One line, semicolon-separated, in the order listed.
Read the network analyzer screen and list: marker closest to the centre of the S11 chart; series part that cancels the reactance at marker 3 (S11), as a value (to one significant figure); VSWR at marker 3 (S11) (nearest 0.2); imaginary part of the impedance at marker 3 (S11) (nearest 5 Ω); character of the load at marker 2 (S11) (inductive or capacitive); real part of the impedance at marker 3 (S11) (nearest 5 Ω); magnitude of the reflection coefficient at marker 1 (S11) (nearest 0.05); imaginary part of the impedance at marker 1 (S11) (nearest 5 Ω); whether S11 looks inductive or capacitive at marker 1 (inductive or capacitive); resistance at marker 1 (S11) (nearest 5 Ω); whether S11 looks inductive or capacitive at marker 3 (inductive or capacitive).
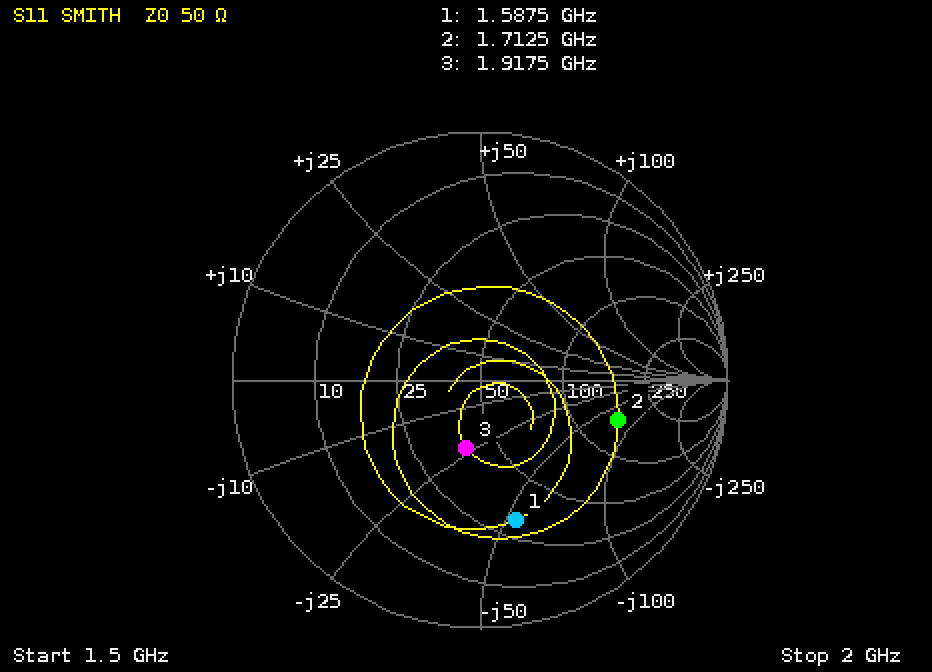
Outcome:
marker 3; 2 nH; 1.8; -25 Ω; capacitive; 40 Ω; 0.60; -55 Ω; capacitive; 30 Ω; capacitive
